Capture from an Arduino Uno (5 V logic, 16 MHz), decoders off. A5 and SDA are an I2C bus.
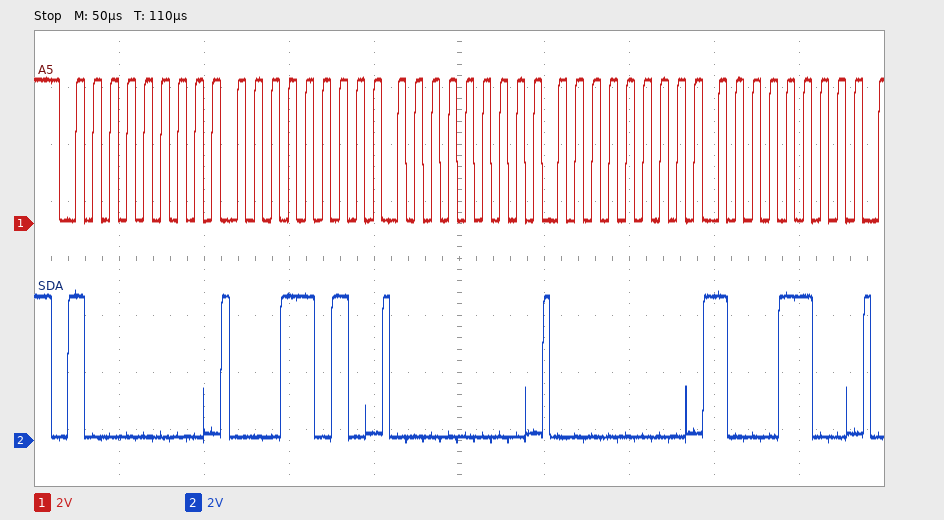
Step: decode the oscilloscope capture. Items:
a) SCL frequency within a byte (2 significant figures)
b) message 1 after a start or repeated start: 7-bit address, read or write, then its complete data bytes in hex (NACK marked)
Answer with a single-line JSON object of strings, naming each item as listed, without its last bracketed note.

{"SCL frequency within a byte": "100 kHz", "message 1 after a start or repeated start: 7-bit address, read or write, then its complete data bytes in hex": "0x40 write: 1A 00 00 8C"}
